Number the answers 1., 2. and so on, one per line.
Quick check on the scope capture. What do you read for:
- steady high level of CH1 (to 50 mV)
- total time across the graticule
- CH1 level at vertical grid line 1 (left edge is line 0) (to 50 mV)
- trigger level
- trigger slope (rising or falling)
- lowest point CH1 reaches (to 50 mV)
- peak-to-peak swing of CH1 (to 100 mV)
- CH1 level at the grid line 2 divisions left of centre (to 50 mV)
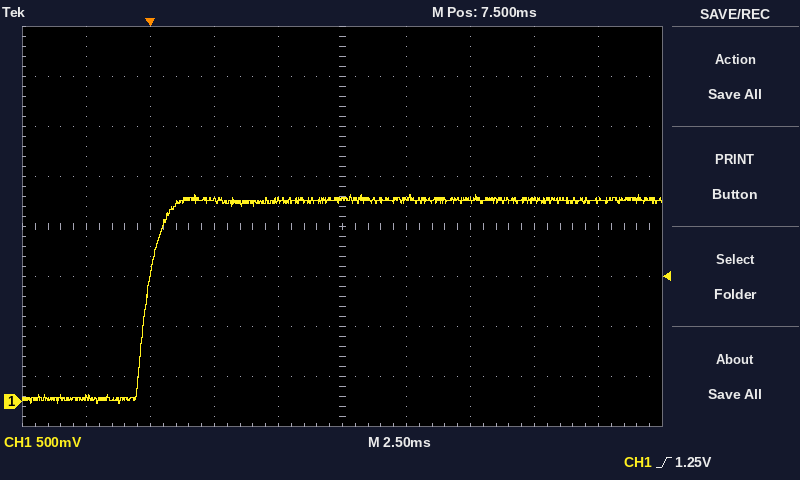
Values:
1. 2.00 V
2. 25 ms
3. 50 mV
4. 1.25 V
5. rising
6. 0 mV
7. 2.10 V
8. 2.00 V
